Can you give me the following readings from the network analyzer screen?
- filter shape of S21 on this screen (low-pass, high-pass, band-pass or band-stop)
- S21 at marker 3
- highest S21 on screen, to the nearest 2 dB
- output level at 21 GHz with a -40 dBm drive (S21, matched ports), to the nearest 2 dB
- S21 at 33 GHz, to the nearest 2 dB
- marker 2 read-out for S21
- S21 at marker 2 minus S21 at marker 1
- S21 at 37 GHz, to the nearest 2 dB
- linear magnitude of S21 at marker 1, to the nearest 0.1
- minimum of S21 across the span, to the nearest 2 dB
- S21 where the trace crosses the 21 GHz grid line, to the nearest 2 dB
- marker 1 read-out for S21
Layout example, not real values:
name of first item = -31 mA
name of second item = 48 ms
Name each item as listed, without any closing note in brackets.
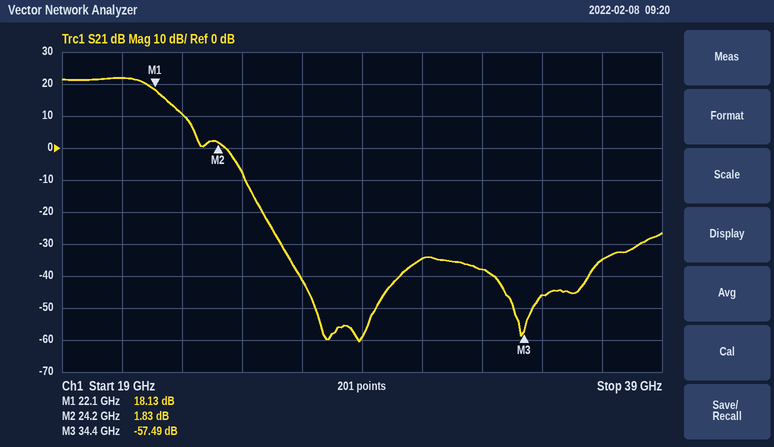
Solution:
filter shape of S21 on this screen = low-pass
S21 at marker 3 = -57.49 dB
highest S21 on screen, to the nearest 2 dB = 22 dB
output level at 21 GHz with a -40 dBm drive (S21, matched ports), to the nearest 2 dB = -18 dBm
S21 at 33 GHz, to the nearest 2 dB = -38 dB
marker 2 read-out for S21 = 1.83 dB
S21 at marker 2 minus S21 at marker 1 = -16.30 dB
S21 at 37 GHz, to the nearest 2 dB = -34 dB
linear magnitude of S21 at marker 1, to the nearest 0.1 = 8.1
minimum of S21 across the span, to the nearest 2 dB = -60 dB
S21 where the trace crosses the 21 GHz grid line, to the nearest 2 dB = 22 dB
marker 1 read-out for S21 = 18.13 dB
